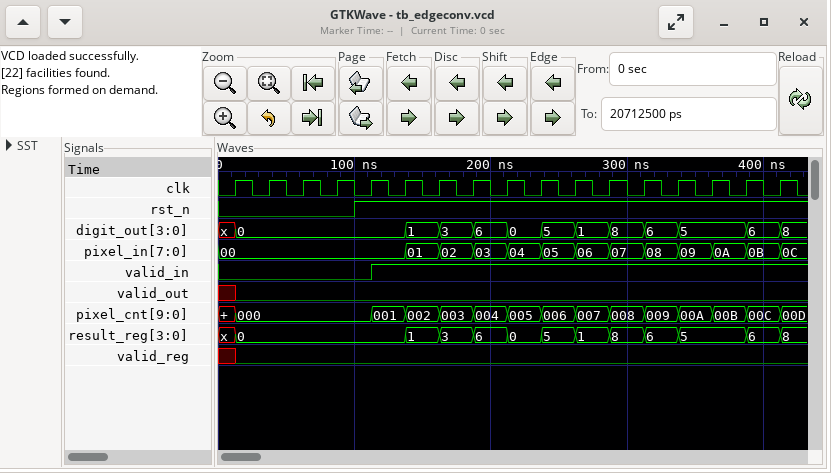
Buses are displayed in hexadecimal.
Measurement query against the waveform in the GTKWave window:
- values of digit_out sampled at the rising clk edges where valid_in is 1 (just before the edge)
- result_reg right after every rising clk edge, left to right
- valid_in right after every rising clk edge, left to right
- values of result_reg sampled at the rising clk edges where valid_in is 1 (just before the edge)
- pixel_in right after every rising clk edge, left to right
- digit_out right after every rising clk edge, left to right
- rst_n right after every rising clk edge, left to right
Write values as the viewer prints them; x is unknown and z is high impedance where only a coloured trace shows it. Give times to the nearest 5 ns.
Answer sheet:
0, 1, 3, 6, 0, 5, 1, 8, 6, 5, 5, 6
0, 0, 0, 0, 0, 1, 3, 6, 0, 5, 1, 8, 6, 5, 5, 6, 8
0 0 0 0 1 1 1 1 1 1 1 1 1 1 1 1 1
0, 1, 3, 6, 0, 5, 1, 8, 6, 5, 5, 6
00, 00, 00, 00, 00, 01, 02, 03, 04, 05, 06, 07, 08, 09, 0A, 0B, 0C
0, 0, 0, 0, 0, 1, 3, 6, 0, 5, 1, 8, 6, 5, 5, 6, 8
0 0 0 0 1 1 1 1 1 1 1 1 1 1 1 1 1
